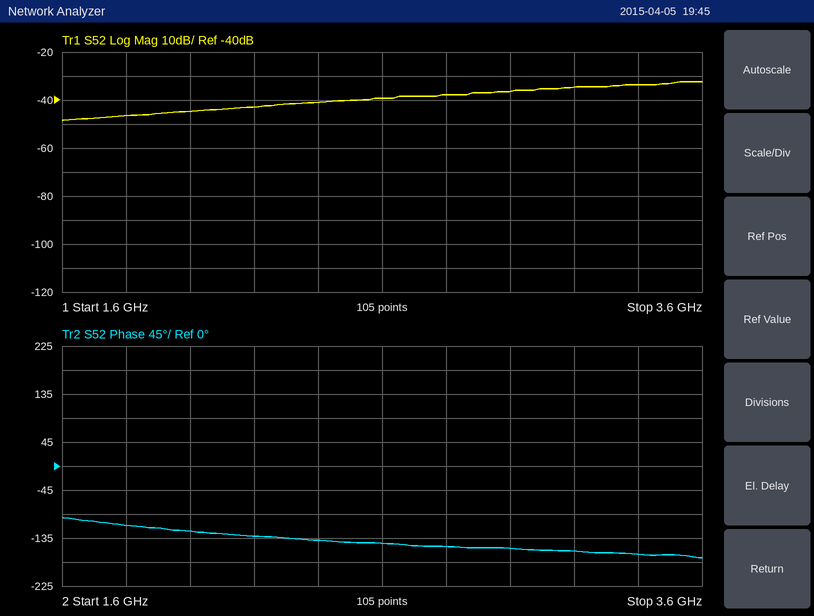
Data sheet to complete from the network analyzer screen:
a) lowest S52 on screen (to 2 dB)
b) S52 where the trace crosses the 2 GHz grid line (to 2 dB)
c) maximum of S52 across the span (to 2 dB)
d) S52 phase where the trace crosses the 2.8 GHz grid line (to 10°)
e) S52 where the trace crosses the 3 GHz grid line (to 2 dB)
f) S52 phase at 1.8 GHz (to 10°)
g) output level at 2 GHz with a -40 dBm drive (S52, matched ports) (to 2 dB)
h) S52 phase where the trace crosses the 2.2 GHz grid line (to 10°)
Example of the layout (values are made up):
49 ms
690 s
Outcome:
-48 dB
-44 dB
-32 dB
-150°
-36 dB
-110°
-84 dBm
-130°
